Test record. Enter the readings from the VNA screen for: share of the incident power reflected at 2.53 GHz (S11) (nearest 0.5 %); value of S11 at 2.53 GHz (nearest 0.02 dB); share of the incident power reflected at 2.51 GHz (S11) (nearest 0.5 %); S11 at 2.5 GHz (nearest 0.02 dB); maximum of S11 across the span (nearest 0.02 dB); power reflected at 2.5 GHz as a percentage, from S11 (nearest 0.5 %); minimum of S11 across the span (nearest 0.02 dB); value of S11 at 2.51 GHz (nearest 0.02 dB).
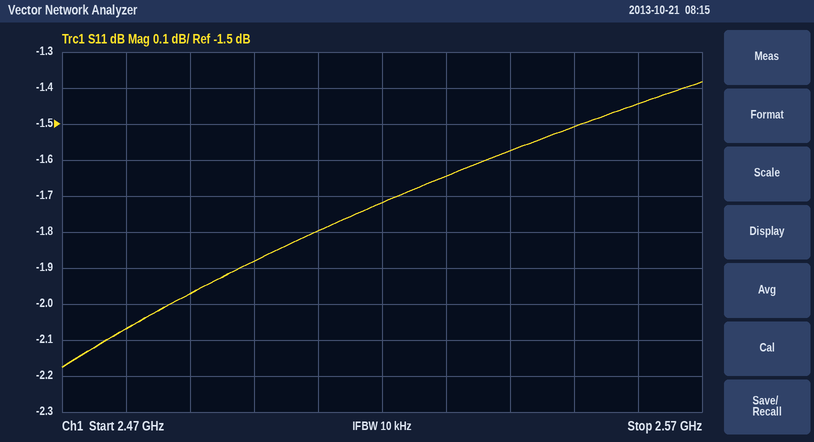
68.5 %
-1.64 dB
66.0 %
-1.88 dB
-1.38 dB
65.0 %
-2.18 dB
-1.80 dB
